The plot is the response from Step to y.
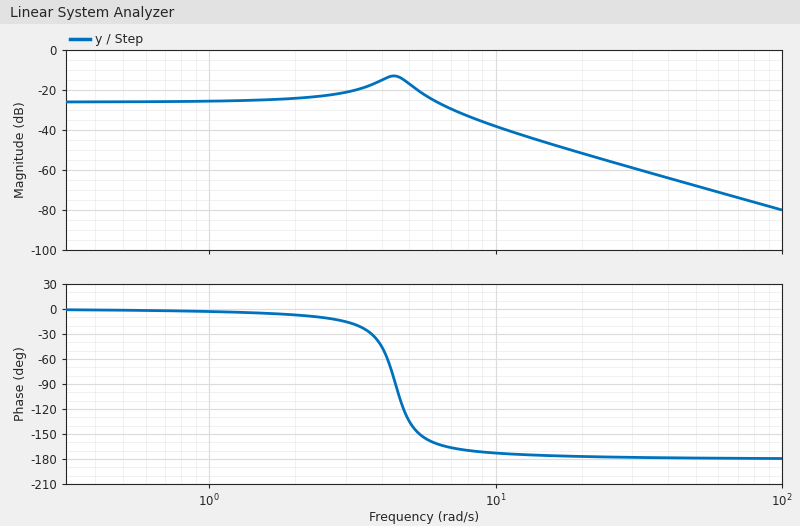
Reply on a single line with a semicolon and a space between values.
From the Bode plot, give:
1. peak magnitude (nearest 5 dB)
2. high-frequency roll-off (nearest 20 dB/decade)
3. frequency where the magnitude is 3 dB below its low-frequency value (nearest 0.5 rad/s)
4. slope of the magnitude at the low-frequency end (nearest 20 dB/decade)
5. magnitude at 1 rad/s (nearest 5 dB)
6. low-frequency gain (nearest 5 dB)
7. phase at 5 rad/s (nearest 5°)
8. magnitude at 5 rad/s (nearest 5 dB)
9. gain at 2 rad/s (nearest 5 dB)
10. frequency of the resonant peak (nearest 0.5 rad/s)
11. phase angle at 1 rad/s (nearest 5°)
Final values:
-15 dB; -40 dB/decade; 7.0 rad/s; 0 dB/decade; -25 dB; -25 dB; -135°; -15 dB; -25 dB; 4.5 rad/s; -5°
